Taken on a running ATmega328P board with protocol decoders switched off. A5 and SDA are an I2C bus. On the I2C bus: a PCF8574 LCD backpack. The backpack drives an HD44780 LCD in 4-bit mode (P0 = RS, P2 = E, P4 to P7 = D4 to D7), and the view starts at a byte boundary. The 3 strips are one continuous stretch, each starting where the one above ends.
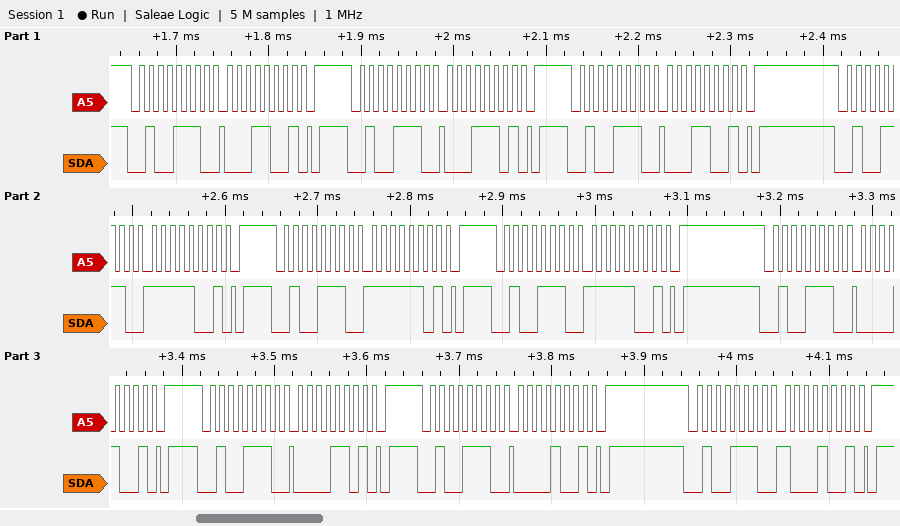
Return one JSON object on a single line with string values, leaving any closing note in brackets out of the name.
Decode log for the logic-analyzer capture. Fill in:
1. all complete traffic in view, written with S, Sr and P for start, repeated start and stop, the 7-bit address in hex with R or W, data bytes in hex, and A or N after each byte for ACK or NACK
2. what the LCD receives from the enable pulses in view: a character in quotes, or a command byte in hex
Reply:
{"all complete traffic in view, written with S, Sr and P for start, repeated start and stop, the 7-bit address in hex with R or W, data bytes in hex, and A or N after each byte for ACK or NACK": "S 27W A 19 A P S 27W A 1D A P S 27W A 19 A P S 27W A F9 A P S 27W A FD A P S 27W A F9 A P S 27W A 09 A P S 27W A 0D A P S 27W A 09 A P S 27W A 89 A P", "what the LCD receives from the enable pulses in view: a character in quotes, or a command byte in hex": "data 0x1F"}
